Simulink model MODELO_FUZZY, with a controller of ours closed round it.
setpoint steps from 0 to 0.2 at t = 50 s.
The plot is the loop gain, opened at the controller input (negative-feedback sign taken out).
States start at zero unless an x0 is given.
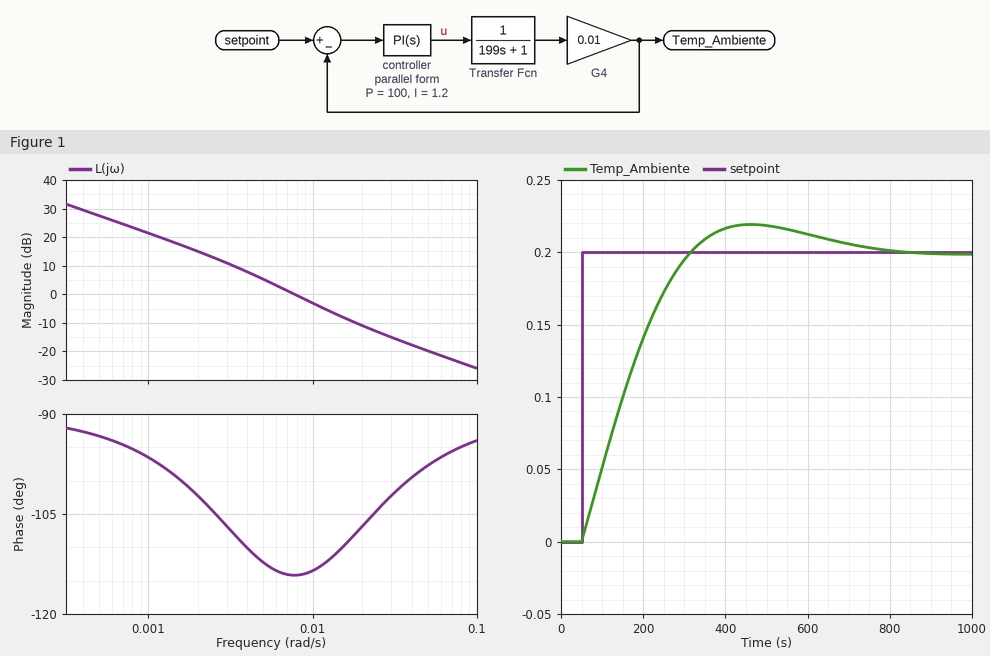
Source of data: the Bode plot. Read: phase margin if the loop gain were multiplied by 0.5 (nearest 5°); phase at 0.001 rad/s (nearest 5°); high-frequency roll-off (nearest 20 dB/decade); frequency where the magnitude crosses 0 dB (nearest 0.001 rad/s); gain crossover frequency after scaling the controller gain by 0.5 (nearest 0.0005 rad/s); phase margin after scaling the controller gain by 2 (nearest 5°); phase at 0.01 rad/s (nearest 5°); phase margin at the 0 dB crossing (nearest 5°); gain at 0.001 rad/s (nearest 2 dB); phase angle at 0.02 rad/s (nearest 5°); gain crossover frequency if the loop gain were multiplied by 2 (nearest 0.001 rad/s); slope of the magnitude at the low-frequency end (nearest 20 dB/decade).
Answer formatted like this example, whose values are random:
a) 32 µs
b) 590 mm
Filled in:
a) 70°
b) -95°
c) -20 dB/decade
d) 0.008 rad/s
e) 0.0045 rad/s
f) 70°
g) -115°
h) 65°
i) 22 dB
j) -105°
k) 0.013 rad/s
l) -20 dB/decade
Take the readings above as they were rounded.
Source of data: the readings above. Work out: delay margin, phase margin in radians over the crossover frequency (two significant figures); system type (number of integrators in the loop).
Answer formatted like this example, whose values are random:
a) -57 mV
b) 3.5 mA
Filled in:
a) 140 s
b) 1
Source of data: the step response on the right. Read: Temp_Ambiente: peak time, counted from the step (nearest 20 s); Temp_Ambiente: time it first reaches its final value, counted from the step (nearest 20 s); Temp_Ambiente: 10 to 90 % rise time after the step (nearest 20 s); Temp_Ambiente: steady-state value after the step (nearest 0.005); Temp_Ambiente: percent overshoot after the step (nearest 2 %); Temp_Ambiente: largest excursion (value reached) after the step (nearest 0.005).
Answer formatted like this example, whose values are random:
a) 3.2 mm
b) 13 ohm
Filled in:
a) 420 s
b) 260 s
c) 200 s
d) 0.200
e) 10 %
f) 0.220
